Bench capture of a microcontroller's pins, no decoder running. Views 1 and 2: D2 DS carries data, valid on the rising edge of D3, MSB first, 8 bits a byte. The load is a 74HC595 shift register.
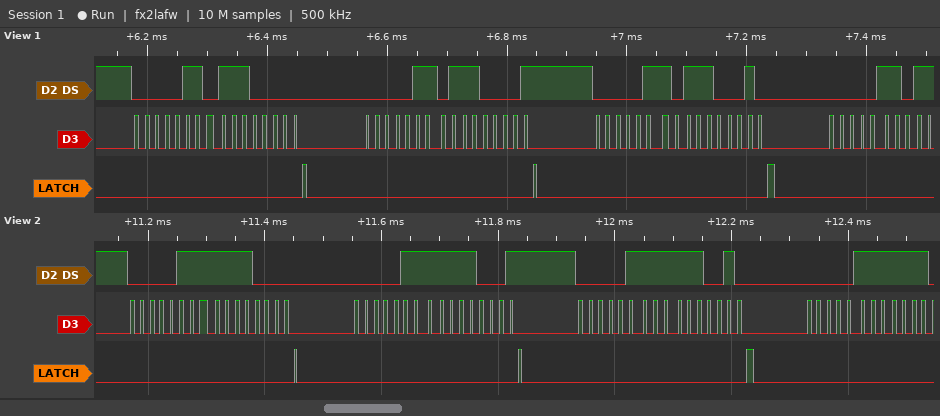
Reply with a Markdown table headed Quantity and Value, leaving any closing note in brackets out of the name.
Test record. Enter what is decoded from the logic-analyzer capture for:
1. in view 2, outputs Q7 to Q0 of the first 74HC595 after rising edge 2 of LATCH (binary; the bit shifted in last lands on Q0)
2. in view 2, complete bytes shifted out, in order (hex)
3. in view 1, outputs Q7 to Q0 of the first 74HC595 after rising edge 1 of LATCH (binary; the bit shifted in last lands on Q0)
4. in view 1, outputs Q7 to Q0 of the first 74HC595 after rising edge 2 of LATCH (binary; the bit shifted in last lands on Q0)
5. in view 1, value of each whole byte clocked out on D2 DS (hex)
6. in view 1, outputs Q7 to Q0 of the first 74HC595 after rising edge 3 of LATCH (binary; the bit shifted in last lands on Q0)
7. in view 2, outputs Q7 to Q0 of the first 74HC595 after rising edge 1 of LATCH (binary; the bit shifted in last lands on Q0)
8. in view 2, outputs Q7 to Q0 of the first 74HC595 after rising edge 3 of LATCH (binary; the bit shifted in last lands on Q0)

| Quantity | Value |
|---|---|
| in view 2, outputs Q7 to Q0 of the first 74HC595 after rising edge 2 of LATCH | 11110001 |
| in view 2, complete bytes shifted out, in order | 0x07 0xF0 0x07 0xF1 0x07 0xF2 0x07 |
| in view 1, outputs Q7 to Q0 of the first 74HC595 after rising edge 1 of LATCH | 11100000 |
| in view 1, outputs Q7 to Q0 of the first 74HC595 after rising edge 2 of LATCH | 11100001 |
| in view 1, value of each whole byte clocked out on D2 DS | 06 E0 06 E1 06 E2 06 |
| in view 1, outputs Q7 to Q0 of the first 74HC595 after rising edge 3 of LATCH | 11100010 |
| in view 2, outputs Q7 to Q0 of the first 74HC595 after rising edge 1 of LATCH | 11110000 |
| in view 2, outputs Q7 to Q0 of the first 74HC595 after rising edge 3 of LATCH | 11110010 |
